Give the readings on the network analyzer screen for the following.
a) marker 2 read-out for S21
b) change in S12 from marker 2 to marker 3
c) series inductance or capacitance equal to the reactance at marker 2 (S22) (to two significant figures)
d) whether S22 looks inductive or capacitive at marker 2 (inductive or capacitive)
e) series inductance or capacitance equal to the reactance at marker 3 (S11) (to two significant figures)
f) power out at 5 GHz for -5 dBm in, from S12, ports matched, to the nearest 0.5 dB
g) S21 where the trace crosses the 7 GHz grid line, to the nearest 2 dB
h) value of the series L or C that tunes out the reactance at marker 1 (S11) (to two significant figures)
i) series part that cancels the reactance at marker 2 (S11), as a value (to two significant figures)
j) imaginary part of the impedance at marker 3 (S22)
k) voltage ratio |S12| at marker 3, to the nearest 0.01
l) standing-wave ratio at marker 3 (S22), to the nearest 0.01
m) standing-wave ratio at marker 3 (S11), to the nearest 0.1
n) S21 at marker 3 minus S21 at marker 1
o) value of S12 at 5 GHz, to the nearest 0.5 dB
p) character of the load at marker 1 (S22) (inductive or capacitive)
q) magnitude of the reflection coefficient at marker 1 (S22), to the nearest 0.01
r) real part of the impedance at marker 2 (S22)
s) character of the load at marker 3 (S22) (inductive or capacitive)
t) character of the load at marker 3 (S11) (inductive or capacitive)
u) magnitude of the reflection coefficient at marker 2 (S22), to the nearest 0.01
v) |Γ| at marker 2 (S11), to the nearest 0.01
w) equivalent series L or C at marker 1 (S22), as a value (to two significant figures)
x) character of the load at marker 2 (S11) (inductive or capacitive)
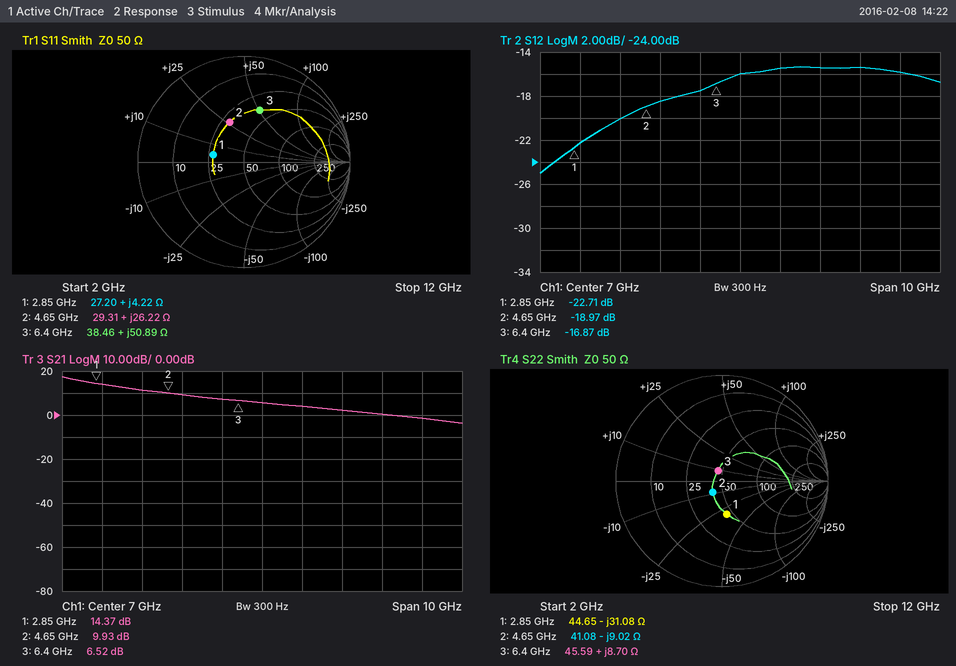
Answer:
9.93 dB
2.10 dB
3.8 pF
capacitive
1.3 nH
-23.5 dBm
6 dB
13 pF
1.3 pF
+8.70 Ω
0.14
1.23
3.1
-7.85 dB
-18.5 dB
capacitive
0.32
41.08 Ω
inductive
inductive
0.14
0.40
1.8 pF
inductive
